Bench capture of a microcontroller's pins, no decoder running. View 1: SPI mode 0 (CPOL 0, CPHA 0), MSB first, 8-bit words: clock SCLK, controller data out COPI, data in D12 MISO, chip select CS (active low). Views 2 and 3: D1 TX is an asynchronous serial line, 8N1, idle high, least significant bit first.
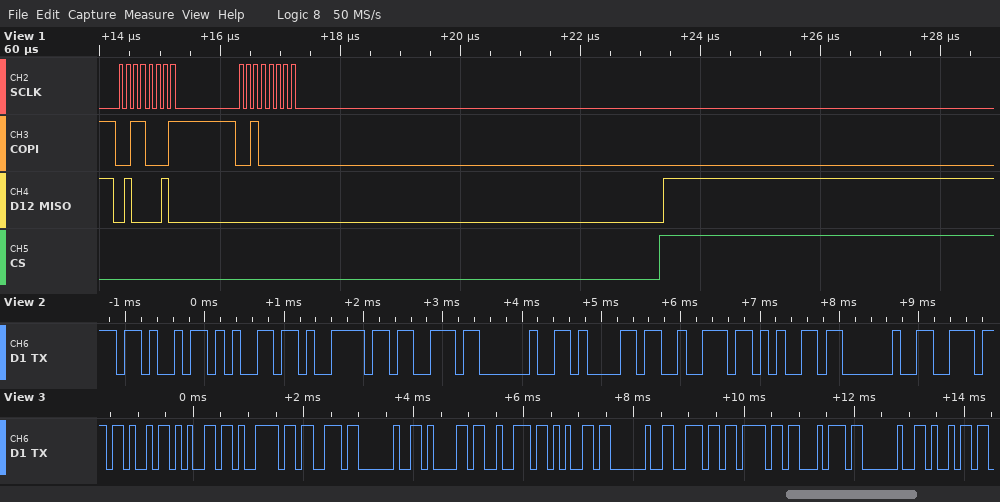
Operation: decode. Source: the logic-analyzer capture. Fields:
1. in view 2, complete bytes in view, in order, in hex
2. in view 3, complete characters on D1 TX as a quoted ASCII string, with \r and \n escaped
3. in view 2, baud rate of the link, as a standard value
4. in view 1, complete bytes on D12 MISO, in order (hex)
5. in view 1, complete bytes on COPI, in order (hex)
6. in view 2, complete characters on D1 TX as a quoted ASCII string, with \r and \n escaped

0x4B 0x65 0x79 0x73 0x20 0x61 0x72 0x65 0x20
"Keys are not i"
9600 baud
42 00
31 20
"Keys are "
